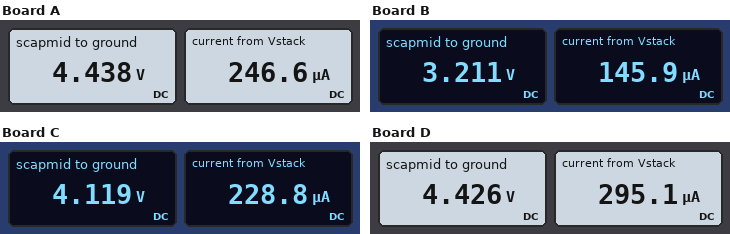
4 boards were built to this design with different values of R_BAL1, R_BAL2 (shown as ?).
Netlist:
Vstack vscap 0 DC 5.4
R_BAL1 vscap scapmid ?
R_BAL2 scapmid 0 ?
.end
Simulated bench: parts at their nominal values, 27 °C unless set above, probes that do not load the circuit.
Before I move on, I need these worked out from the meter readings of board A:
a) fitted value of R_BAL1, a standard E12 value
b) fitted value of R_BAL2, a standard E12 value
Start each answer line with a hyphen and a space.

- 3.9 kΩ
- 18 kΩ
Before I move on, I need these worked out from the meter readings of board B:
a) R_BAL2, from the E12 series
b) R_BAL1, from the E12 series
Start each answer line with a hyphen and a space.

- 22 kΩ
- 15 kΩ
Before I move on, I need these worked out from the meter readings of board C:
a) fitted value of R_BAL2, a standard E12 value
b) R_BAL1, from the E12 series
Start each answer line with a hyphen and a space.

- 18 kΩ
- 5.6 kΩ
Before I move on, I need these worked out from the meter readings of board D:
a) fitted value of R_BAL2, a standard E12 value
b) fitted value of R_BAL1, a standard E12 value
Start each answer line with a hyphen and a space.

- 15 kΩ
- 3.3 kΩ
